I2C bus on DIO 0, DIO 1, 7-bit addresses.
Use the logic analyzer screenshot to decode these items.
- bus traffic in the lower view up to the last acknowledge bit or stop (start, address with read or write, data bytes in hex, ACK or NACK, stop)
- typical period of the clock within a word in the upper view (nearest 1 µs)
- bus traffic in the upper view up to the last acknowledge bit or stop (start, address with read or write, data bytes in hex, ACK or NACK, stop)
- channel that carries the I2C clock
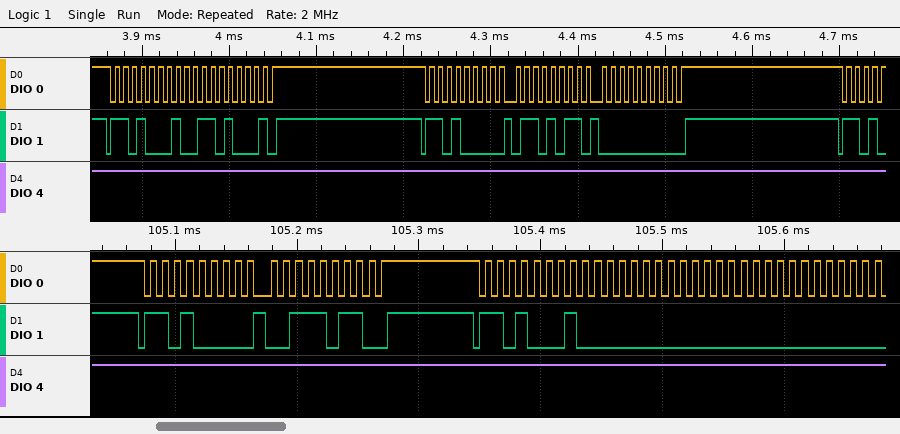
start, address 68 write ACK, 3B ACK, stop, start, address 68 read ACK, 00 ACK, 00 ACK
10 µs
start, address 68 read ACK, 68 NACK, stop, start, address 68 write ACK, 6B ACK, 00 ACK, stop
DIO 0
